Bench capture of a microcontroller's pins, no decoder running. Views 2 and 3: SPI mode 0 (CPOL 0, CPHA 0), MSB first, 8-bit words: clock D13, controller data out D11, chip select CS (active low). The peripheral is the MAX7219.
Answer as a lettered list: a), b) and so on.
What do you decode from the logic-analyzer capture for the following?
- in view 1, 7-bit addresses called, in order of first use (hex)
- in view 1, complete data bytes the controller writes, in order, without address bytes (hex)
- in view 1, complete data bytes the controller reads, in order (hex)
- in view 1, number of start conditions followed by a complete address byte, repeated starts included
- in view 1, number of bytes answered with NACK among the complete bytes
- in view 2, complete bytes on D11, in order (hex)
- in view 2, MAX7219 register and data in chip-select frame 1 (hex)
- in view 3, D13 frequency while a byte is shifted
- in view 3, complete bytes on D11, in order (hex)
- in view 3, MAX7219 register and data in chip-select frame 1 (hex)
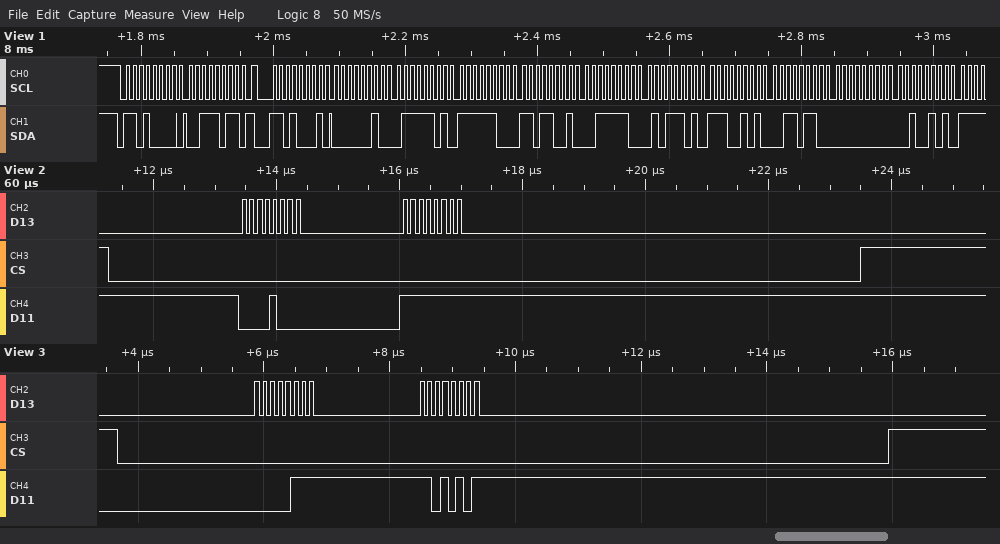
a) 0x68
b) 3B
c) 02 7D FC D9 3E 5D E5 36 00 25
d) 2
e) 0
f) 08 FF
g) register 0x8, data 0xFF
h) 8 MHz
i) 07 D5
j) register 0x7, data 0xD5
